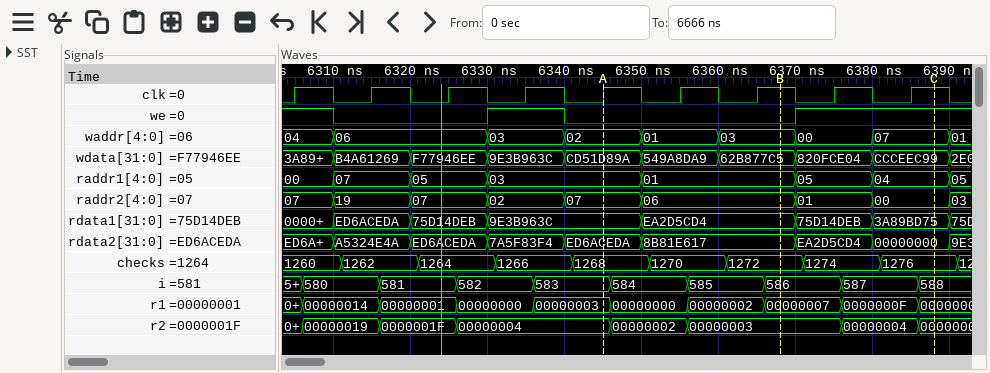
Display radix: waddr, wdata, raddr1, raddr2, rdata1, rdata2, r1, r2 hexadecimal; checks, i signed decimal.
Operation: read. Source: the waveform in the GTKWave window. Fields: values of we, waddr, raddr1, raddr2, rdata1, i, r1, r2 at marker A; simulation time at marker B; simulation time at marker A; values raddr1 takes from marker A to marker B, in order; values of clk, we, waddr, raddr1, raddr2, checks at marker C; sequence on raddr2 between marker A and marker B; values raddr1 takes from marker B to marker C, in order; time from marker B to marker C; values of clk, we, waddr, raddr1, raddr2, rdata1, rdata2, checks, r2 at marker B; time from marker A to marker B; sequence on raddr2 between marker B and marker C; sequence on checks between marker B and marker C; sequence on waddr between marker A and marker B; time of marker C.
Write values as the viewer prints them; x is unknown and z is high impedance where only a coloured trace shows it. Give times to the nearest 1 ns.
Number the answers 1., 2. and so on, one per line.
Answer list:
1. we=0, waddr=02, raddr1=03, raddr2=07, rdata1=9E3B963C, i=583, r1=00000003, r2=00000004
2. 6368 ns
3. 6345 ns
4. 03, 01
5. clk=1, we=1, waddr=07, raddr1=04, raddr2=00, checks=1276
6. 07, 06
7. 01, 05, 04
8. 20 ns
9. clk=1, we=0, waddr=03, raddr1=01, raddr2=06, rdata1=EA2D5CD4, rdata2=8B81E617, checks=1272, r2=00000003
10. 23 ns
11. 06, 01, 00
12. 1272, 1274, 1276
13. 02, 01, 03
14. 6388 ns
